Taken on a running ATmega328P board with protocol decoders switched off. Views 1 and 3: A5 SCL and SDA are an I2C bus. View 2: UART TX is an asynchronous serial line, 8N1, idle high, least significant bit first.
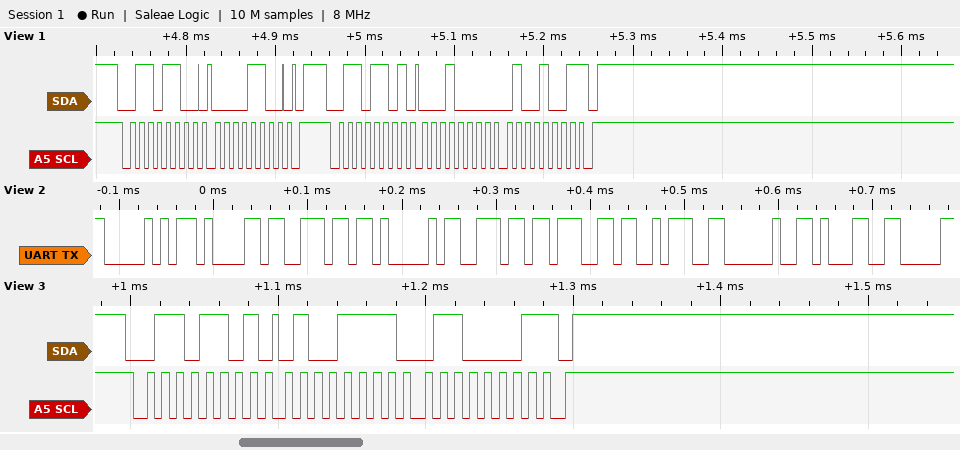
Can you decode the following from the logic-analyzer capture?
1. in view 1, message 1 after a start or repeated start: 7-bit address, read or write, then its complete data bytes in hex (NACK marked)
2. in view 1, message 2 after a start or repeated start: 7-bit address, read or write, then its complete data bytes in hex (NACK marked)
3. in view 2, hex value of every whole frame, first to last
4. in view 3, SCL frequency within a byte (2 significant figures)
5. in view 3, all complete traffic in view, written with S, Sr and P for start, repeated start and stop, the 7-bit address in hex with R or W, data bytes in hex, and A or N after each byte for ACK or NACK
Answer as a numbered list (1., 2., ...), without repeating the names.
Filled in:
1. 0x36 write: 0C
2. 0x36 read: 10 49 NACK
3. 50 61 6E 41 6E 67 3A 20 31
4. 100 kHz
5. S 36R A 4F A 61 N P
